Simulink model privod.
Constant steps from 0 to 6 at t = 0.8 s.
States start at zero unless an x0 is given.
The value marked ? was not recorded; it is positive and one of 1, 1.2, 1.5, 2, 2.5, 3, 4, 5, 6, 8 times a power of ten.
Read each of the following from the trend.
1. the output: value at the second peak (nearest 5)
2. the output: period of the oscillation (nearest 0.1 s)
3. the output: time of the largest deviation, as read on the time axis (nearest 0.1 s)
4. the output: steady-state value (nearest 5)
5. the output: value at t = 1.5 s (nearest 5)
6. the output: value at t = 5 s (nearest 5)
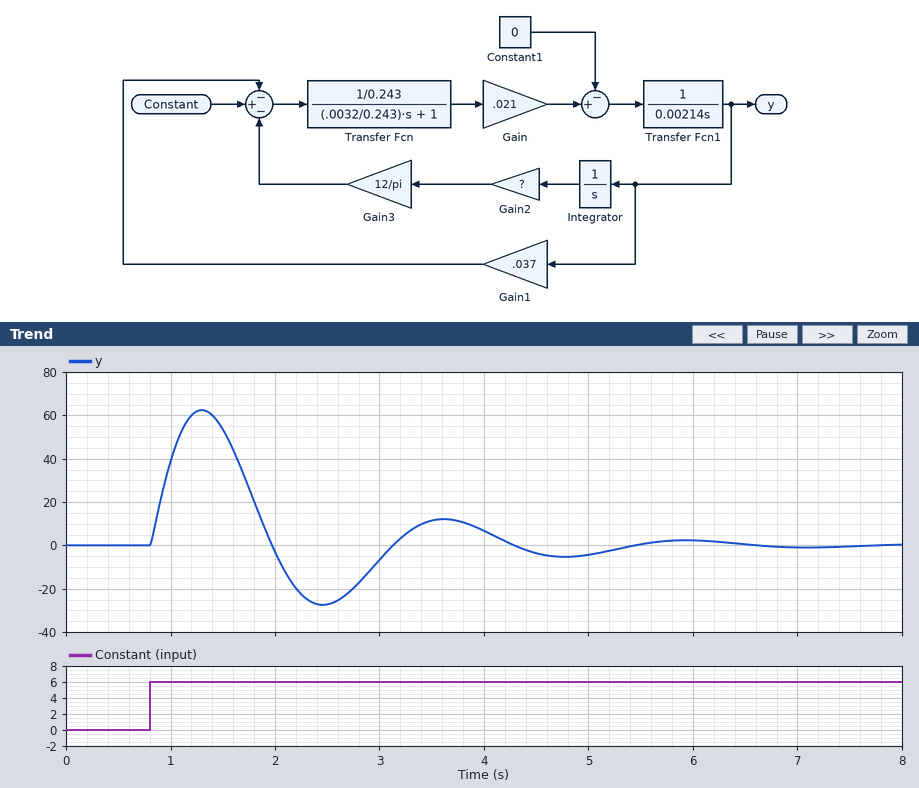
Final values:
10
2.3 s
1.3 s
0
55
-5
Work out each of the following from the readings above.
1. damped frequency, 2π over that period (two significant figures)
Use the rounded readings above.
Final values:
2.7 rad/s
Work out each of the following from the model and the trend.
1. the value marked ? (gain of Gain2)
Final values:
0.05
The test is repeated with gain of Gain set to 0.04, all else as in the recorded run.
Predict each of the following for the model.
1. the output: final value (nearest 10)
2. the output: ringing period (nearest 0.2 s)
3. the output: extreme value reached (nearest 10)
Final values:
0
1.8 s
80
